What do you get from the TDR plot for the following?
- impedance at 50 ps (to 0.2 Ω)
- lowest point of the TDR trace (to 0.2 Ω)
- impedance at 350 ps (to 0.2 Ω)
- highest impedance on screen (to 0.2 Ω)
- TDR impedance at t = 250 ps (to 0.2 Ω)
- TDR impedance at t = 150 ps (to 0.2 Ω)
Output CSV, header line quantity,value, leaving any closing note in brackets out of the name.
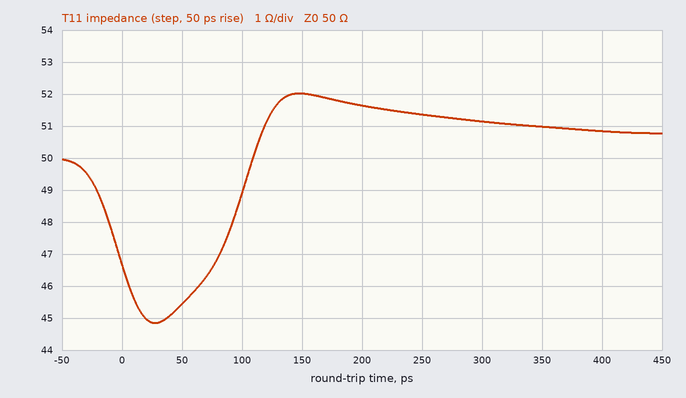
quantity,value
impedance at 50 ps,45.4 Ω
lowest point of the TDR trace,44.8 Ω
impedance at 350 ps,51.0 Ω
highest impedance on screen,52.0 Ω
TDR impedance at t = 250 ps,51.4 Ω
TDR impedance at t = 150 ps,52.0 Ω
